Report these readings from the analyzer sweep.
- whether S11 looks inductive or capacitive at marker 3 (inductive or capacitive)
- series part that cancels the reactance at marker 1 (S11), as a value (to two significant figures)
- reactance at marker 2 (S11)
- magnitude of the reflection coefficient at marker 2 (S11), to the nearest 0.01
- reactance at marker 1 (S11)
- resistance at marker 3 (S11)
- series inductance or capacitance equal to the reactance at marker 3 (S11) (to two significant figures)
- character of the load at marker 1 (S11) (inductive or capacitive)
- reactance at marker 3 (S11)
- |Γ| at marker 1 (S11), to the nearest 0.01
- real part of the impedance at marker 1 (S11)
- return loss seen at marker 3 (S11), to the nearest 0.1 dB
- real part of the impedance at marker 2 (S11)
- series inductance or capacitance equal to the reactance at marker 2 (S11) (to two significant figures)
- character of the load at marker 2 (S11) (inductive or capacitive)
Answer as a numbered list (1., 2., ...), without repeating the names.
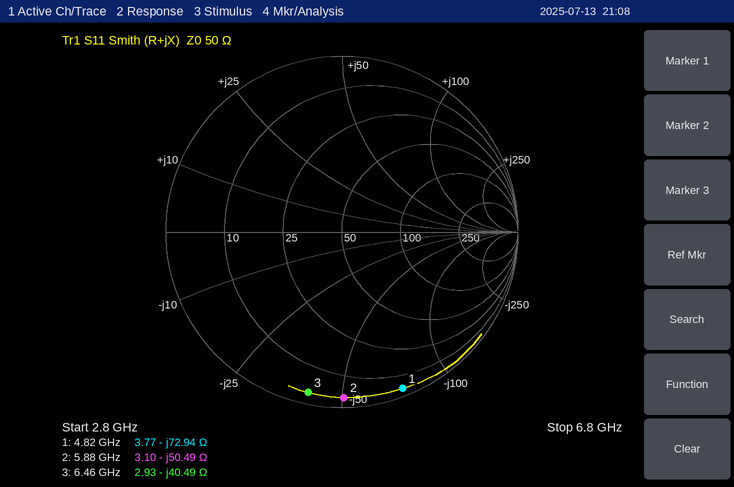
1. capacitive
2. 2.4 nH
3. -50.49 Ω
4. 0.94
5. -72.94 Ω
6. 2.93 Ω
7. 610 fF
8. capacitive
9. -40.49 Ω
10. 0.95
11. 3.77 Ω
12. 0.6 dB
13. 3.10 Ω
14. 540 fF
15. capacitive
